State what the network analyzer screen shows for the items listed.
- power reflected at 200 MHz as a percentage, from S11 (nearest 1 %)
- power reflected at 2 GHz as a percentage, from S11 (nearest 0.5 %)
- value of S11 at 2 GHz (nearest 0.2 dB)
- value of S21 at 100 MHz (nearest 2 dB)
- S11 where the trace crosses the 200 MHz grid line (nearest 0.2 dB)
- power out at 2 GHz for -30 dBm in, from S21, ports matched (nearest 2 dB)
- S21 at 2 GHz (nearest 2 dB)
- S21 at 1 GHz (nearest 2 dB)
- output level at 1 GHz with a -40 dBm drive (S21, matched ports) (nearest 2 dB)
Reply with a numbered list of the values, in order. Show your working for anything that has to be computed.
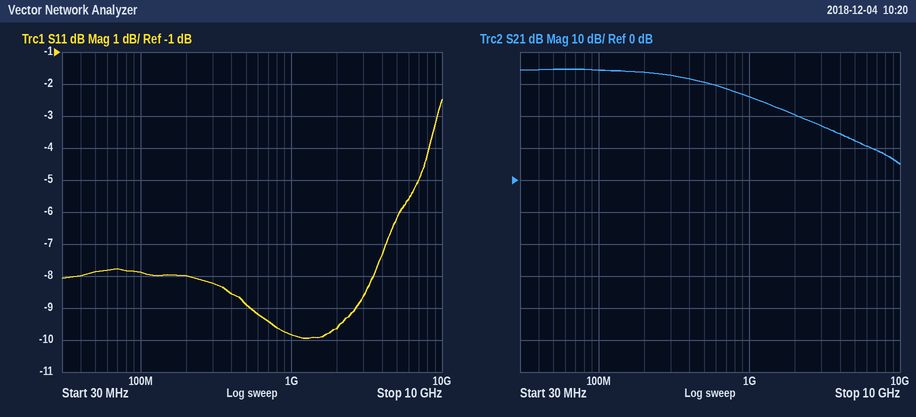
1. 10^(-8/10) ≈ 16 %
2. 10^(-9.6/10) ≈ 11.0 %
3. -9.6 dB
4. 34 dB
5. -8.0 dB
6. -30 dBm + (20 dB) = -10 dBm
7. 20 dB
8. 26 dB
9. -40 dBm + (26 dB) = -14 dBm
